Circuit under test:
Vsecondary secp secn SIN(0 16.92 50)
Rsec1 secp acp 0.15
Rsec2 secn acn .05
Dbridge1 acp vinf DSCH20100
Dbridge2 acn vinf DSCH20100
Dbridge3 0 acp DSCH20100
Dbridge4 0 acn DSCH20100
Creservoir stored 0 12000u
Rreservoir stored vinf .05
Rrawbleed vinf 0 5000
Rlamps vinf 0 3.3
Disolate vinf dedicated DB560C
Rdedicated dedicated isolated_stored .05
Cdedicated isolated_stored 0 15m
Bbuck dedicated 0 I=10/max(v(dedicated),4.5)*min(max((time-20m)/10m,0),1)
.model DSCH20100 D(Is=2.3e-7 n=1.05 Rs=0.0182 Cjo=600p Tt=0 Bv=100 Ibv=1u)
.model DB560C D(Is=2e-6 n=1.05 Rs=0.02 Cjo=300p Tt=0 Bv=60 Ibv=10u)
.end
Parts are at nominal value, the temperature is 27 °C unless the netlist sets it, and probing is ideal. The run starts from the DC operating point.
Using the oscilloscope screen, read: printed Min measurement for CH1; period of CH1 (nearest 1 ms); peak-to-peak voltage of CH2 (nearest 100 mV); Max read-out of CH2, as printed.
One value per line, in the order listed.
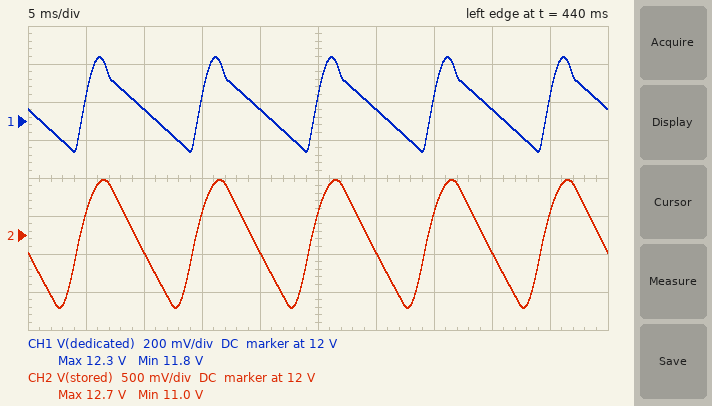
11.8 V
10 ms
1.7 V
12.7 V
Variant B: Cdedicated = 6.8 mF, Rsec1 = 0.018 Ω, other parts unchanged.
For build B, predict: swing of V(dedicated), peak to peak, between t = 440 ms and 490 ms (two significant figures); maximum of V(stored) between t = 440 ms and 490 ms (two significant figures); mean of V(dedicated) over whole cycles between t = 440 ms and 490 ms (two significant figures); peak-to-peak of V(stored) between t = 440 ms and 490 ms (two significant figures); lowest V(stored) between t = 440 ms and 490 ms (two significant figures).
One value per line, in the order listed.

900 mV
14 V
13 V
2.1 V
12 V
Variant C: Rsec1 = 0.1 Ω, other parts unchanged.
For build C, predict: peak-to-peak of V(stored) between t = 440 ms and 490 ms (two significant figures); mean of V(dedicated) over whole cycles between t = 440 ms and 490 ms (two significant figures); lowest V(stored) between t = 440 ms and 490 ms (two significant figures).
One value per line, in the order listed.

1.8 V
13 V
11 V
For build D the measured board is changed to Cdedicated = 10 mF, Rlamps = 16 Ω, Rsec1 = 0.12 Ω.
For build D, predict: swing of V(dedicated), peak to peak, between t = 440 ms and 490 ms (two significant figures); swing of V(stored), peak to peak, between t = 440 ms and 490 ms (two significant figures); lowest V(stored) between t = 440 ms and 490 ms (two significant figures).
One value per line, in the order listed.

510 mV
570 mV
14 V
